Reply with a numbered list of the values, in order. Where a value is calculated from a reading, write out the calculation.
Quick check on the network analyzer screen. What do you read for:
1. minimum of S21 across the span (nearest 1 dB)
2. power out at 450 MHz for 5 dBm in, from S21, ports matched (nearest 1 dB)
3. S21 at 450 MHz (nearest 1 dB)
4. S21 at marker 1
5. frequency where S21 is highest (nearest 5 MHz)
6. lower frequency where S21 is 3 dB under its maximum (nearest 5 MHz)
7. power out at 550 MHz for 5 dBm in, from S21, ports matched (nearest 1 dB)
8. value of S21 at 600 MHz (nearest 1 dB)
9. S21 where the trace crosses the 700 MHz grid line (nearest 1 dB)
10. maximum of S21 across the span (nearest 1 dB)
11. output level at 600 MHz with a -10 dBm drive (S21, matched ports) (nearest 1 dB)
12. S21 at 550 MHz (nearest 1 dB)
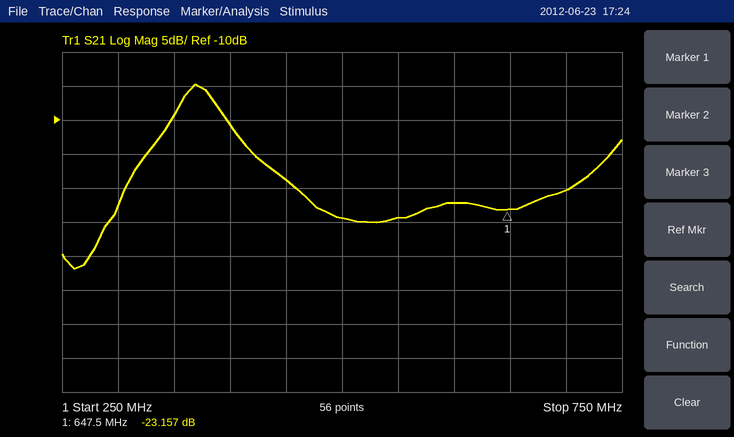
1. -32 dB
2. 5 dBm + (-19 dB) = -14 dBm
3. -19 dB
4. -23.157 dB
5. 370 MHz
6. 355 MHz
7. 5 dBm + (-24 dB) = -19 dBm
8. -22 dB
9. -20 dB
10. -5 dB
11. -10 dBm + (-22 dB) = -32 dBm
12. -24 dB
